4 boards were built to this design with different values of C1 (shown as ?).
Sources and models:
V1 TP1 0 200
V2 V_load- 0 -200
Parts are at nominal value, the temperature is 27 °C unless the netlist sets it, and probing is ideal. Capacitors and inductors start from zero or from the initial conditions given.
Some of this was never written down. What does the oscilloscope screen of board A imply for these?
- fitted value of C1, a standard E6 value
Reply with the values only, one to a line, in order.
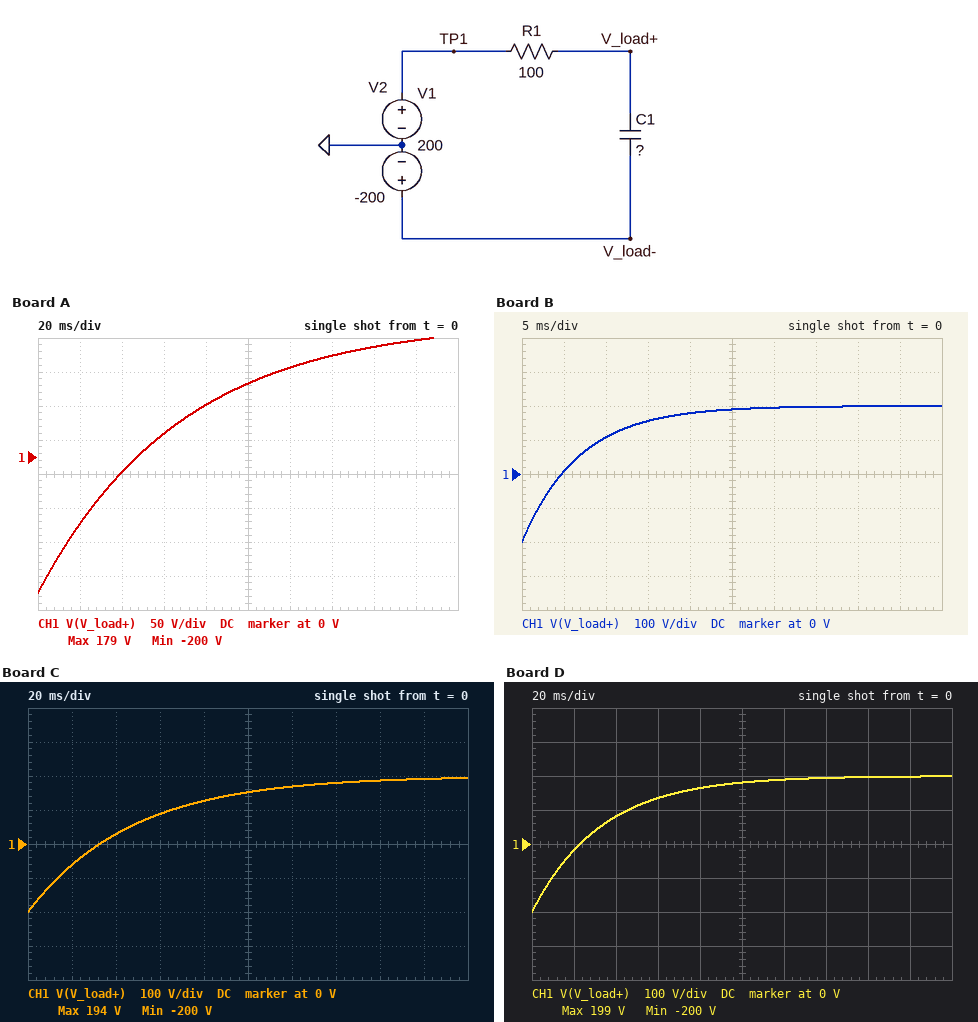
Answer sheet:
680 µF
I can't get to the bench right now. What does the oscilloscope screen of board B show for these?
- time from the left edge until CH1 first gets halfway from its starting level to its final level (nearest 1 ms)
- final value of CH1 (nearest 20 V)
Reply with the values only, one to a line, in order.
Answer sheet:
5 ms
200 V
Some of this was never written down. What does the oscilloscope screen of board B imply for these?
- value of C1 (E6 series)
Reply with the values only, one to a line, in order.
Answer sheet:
68 µF
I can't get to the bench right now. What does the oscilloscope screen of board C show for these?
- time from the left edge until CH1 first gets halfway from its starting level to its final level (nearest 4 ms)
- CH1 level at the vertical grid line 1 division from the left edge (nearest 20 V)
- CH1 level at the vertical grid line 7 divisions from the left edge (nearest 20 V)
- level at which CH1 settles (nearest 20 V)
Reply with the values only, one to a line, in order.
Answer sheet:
32 ms
-60 V
180 V
200 V
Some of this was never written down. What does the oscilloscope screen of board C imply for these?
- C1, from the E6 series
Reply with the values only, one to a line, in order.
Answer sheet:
470 µF
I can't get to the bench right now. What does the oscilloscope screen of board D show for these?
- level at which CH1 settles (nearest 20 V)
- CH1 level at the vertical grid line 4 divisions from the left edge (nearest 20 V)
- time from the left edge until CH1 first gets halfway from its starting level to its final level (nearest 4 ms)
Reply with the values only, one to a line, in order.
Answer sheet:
200 V
160 V
24 ms
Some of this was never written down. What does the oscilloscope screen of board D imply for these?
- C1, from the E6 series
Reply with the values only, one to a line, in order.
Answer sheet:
330 µF
